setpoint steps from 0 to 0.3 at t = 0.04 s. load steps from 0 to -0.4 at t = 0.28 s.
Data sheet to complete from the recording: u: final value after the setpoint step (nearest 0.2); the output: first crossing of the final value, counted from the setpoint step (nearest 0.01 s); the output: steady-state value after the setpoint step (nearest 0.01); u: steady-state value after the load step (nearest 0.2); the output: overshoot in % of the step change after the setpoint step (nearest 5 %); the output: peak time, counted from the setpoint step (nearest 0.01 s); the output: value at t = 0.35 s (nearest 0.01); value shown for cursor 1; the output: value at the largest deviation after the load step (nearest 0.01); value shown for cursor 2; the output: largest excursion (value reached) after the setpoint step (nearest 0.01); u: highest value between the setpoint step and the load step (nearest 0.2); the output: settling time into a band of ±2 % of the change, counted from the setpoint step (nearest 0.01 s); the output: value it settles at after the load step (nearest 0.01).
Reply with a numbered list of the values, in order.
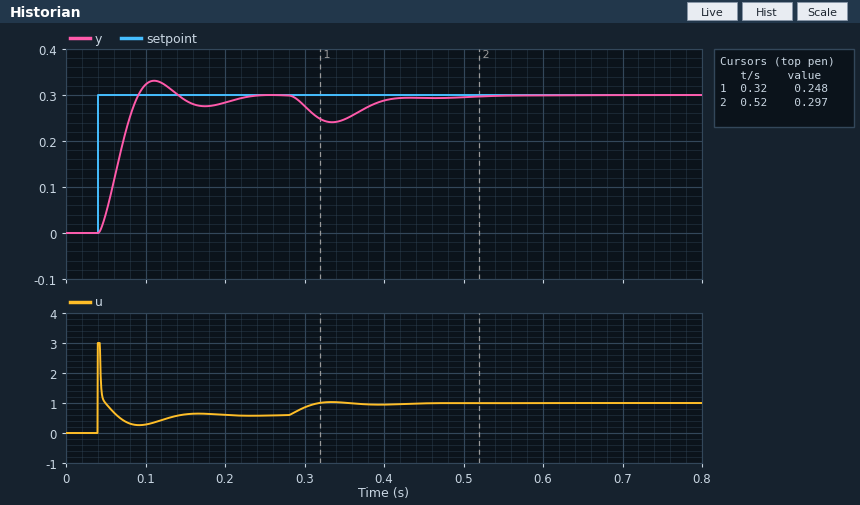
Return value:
1. 0.6
2. 0.05 s
3. 0.30
4. 1.0
5. 10 %
6. 0.07 s
7. 0.25
8. 0.248
9. 0.24
10. 0.297
11. 0.33
12. 3.0
13. 0.18 s
14. 0.30
